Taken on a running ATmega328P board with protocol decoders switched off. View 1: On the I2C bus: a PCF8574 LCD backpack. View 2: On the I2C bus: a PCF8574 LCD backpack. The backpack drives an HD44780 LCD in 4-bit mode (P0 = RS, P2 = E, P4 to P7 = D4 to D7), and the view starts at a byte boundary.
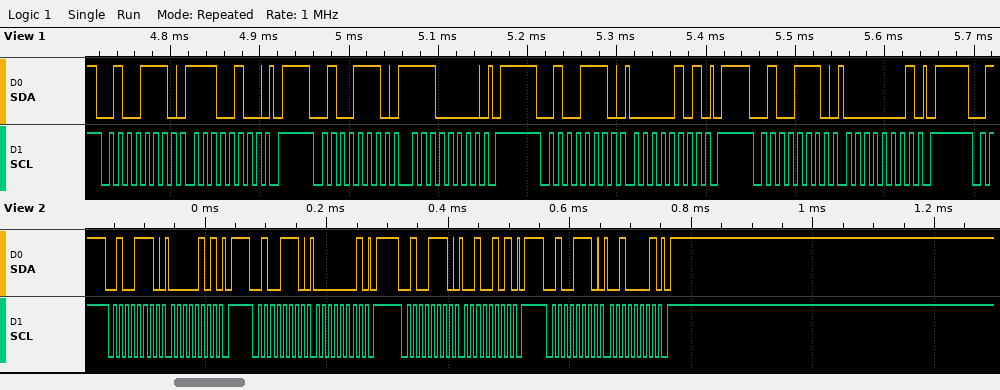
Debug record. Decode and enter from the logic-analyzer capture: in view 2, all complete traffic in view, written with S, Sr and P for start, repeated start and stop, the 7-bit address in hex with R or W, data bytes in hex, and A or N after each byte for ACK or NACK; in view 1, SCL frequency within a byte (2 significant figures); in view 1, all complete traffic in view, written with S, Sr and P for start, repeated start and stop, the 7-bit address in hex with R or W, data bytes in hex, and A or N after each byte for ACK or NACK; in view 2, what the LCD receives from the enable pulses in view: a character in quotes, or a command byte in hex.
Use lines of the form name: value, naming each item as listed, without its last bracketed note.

in view 2, all complete traffic in view, written with S, Sr and P for start, repeated start and stop, the 7-bit address in hex with R or W, data bytes in hex, and A or N after each byte for ACK or NACK: S 27W A 05 A P S 27W A 01 A P S 27W A 25 A P S 27W A 21 A P
in view 1, SCL frequency within a byte: 100 kHz
in view 1, all complete traffic in view, written with S, Sr and P for start, repeated start and stop, the 7-bit address in hex with R or W, data bytes in hex, and A or N after each byte for ACK or NACK: S 27W A E4 A P S 27W A E0 A P S 27W A 05 A P S 27W A 01 A P
in view 2, what the LCD receives from the enable pulses in view: a character in quotes, or a command byte in hex: data 0x02
